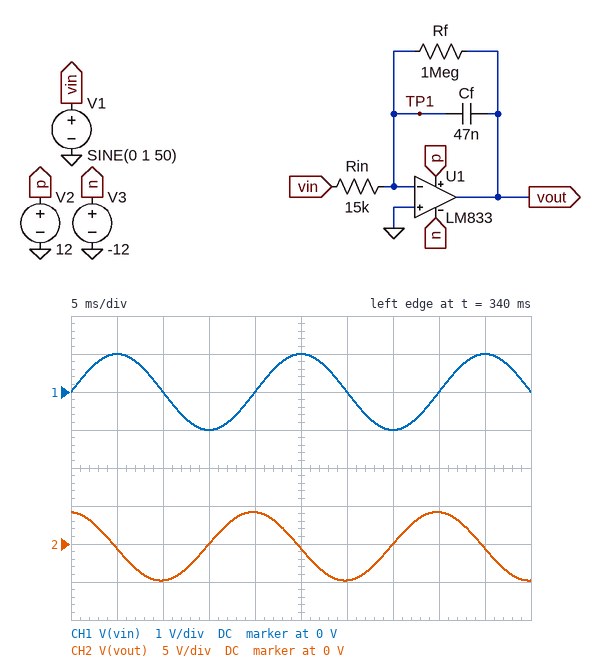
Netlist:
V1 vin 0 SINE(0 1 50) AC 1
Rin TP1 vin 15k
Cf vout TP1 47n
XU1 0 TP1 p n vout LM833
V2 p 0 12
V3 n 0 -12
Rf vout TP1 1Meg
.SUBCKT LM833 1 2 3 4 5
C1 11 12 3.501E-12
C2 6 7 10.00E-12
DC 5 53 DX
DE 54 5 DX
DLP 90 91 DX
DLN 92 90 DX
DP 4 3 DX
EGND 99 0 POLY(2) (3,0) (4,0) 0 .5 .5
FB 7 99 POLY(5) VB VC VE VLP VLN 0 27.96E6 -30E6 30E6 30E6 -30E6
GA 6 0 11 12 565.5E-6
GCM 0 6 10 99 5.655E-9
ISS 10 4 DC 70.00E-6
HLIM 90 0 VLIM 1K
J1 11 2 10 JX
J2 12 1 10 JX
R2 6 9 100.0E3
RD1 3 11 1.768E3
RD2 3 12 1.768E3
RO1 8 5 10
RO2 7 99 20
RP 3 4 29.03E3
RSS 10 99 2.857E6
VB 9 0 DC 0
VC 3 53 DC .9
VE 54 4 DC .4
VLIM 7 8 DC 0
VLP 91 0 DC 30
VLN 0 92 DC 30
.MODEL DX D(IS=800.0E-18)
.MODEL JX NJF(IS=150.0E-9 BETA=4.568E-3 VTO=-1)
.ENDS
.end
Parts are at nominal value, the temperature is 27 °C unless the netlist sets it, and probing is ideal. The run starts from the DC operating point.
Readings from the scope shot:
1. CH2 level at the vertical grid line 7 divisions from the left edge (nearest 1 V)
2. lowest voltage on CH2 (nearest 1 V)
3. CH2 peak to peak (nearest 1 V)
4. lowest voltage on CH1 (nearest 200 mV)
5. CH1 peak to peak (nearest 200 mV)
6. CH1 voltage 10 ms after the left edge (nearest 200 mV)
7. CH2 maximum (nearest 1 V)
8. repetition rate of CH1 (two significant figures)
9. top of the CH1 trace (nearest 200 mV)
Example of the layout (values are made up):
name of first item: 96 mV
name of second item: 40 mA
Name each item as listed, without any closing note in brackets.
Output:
CH2 level at the vertical grid line 7 divisions from the left edge: 0 V
lowest voltage on CH2: -5 V
CH2 peak to peak: 9 V
lowest voltage on CH1: -1.0 V
CH1 peak to peak: 2.0 V
CH1 voltage 10 ms after the left edge: 0 V
CH2 maximum: 4 V
repetition rate of CH1: 50 Hz
top of the CH1 trace: 1.0 V
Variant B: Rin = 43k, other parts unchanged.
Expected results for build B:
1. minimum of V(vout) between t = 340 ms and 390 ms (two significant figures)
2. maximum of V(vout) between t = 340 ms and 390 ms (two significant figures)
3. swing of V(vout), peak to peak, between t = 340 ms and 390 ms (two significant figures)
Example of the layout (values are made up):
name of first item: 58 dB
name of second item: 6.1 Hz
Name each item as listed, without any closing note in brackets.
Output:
minimum of V(vout) between t = 340 ms and 390 ms: -1.9 V
maximum of V(vout) between t = 340 ms and 390 ms: 1.3 V
swing of V(vout), peak to peak, between t = 340 ms and 390 ms: 3.1 V
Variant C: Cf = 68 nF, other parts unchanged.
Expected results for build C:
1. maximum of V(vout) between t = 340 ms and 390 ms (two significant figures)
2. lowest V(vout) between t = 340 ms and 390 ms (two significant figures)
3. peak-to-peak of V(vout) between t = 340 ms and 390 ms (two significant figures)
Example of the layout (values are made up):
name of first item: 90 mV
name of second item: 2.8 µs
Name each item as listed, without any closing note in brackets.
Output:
maximum of V(vout) between t = 340 ms and 390 ms: 2.8 V
lowest V(vout) between t = 340 ms and 390 ms: -3.4 V
peak-to-peak of V(vout) between t = 340 ms and 390 ms: 6.2 V
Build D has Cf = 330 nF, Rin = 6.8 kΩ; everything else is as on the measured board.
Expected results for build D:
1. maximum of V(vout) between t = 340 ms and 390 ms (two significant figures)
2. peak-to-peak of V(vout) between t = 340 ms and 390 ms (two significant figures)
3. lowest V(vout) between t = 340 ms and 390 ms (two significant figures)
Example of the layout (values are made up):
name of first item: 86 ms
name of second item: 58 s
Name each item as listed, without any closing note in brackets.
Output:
maximum of V(vout) between t = 340 ms and 390 ms: 670 mV
peak-to-peak of V(vout) between t = 340 ms and 390 ms: 2.9 V
lowest V(vout) between t = 340 ms and 390 ms: -2.2 V
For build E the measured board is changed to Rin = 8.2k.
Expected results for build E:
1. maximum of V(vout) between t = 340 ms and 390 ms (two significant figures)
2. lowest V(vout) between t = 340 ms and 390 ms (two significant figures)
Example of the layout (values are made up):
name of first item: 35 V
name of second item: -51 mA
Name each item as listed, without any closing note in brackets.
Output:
maximum of V(vout) between t = 340 ms and 390 ms: 7.9 V
lowest V(vout) between t = 340 ms and 390 ms: -8.5 V
